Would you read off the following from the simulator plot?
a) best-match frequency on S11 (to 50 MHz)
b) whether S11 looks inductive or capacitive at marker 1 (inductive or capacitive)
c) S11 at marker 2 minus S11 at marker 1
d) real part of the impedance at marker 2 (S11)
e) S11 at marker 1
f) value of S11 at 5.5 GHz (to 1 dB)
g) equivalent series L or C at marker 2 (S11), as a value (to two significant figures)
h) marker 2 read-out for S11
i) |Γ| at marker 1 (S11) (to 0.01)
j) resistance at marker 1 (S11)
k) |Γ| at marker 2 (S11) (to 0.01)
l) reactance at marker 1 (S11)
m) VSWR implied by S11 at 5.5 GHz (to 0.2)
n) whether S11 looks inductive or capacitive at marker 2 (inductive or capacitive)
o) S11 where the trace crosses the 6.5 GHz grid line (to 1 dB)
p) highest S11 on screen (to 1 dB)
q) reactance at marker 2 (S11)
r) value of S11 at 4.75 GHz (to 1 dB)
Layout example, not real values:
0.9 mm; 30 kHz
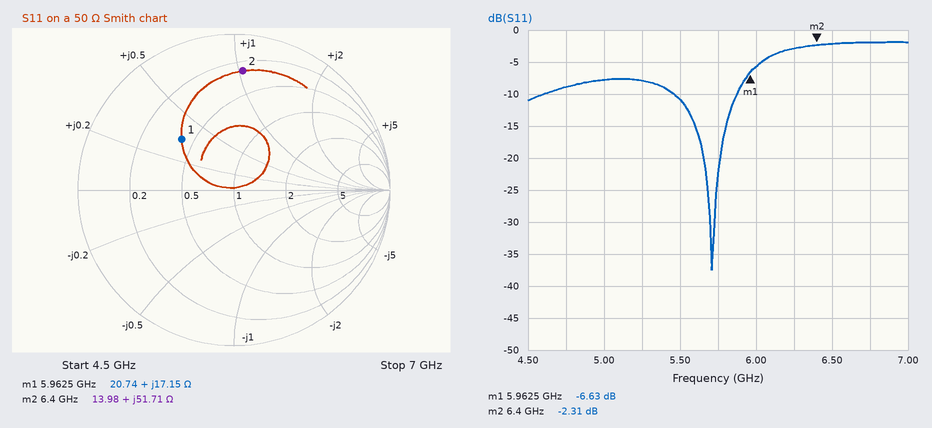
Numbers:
5.70 GHz; inductive; 4.32 dB; 13.98 Ω; -6.63 dB; -11 dB; 1.3 nH; -2.31 dB; 0.47; 20.74 Ω; 0.77; +17.15 Ω; 1.8; inductive; -2 dB; -2 dB; +51.71 Ω; -9 dB
